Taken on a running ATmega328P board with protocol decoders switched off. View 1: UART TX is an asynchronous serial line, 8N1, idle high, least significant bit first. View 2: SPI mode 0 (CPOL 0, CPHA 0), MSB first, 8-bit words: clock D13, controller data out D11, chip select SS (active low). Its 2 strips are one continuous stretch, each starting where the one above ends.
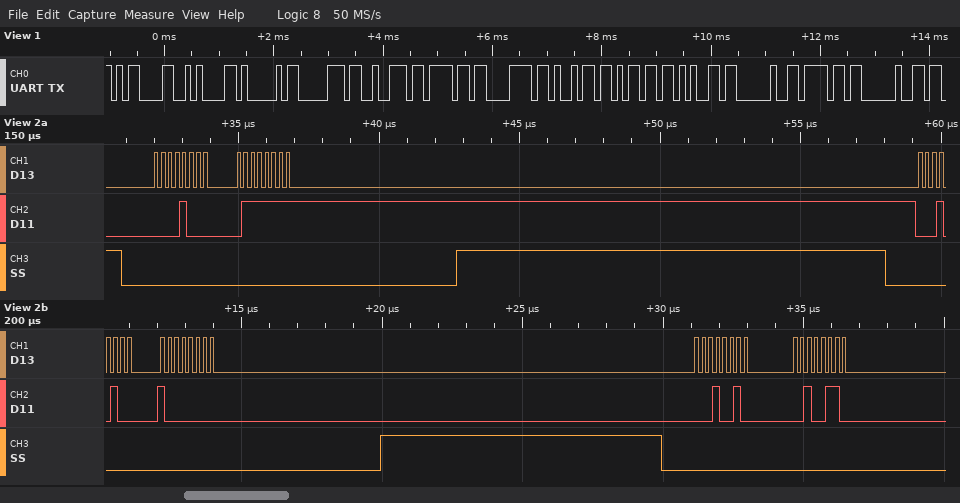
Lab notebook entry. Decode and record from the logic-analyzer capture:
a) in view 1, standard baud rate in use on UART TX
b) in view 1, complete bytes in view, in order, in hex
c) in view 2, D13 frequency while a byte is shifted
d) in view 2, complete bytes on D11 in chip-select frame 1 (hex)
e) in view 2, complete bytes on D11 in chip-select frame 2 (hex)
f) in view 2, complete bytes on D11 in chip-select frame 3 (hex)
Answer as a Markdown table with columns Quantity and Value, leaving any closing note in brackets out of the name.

| Quantity | Value |
|---|---|
| in view 1, standard baud rate in use on UART TX | 9600 baud |
| in view 1, complete bytes in view, in order, in hex | 0x0D 0x0A 0x41 0x70 0x72 0x6F 0x78 0x69 0x6D 0x65 0x20 0x6F 0x20 |
| in view 2, D13 frequency while a byte is shifted | 4 MHz |
| in view 2, complete bytes on D11 in chip-select frame 1 | 08 7F |
| in view 2, complete bytes on D11 in chip-select frame 2 | 14 80 |
| in view 2, complete bytes on D11 in chip-select frame 3 | 12 26 |
